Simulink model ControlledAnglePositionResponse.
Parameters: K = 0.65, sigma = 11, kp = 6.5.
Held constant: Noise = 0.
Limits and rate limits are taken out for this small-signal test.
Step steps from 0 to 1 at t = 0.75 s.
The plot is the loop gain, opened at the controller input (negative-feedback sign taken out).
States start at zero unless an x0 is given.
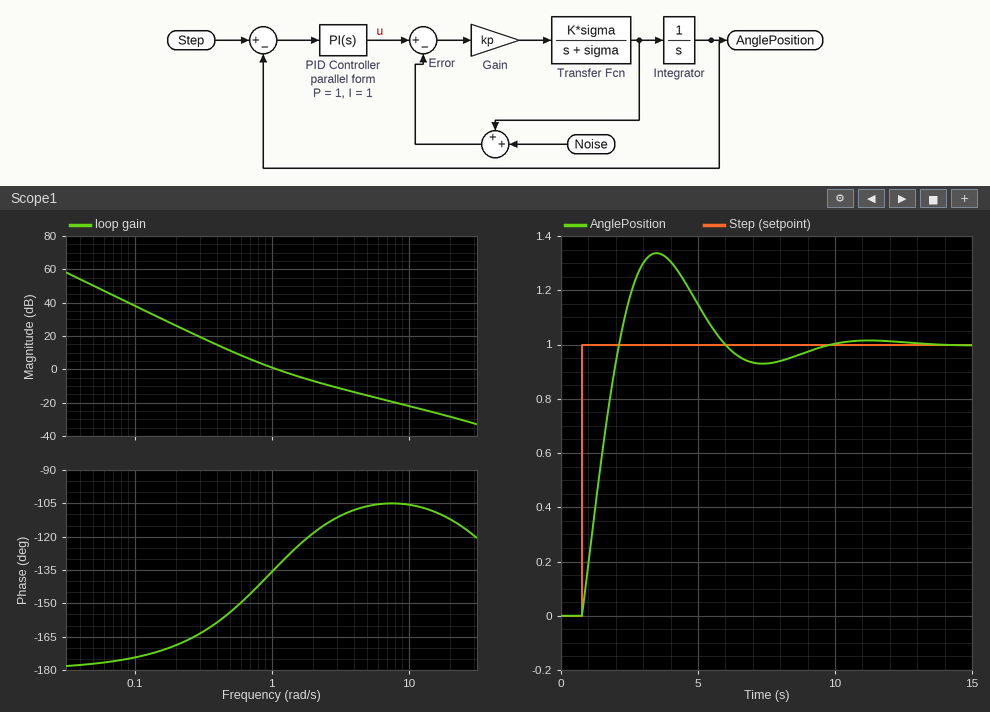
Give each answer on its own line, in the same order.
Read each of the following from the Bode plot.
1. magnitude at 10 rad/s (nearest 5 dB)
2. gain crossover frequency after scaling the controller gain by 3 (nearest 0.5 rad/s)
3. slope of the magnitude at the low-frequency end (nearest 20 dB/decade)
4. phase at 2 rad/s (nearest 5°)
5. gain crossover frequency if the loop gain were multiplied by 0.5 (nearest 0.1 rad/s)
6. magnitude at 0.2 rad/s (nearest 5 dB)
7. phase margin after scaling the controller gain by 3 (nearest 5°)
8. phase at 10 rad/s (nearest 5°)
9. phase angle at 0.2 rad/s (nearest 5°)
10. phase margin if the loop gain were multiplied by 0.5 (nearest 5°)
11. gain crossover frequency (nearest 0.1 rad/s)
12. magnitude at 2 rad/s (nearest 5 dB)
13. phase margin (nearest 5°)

-20 dB
2.5 rad/s
-40 dB/decade
-120°
0.7 rad/s
25 dB
65°
-105°
-170°
35°
1.1 rad/s
-5 dB
45°
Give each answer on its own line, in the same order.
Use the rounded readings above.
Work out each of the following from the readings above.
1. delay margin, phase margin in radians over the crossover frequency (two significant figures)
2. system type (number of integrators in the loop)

0.71 s
2
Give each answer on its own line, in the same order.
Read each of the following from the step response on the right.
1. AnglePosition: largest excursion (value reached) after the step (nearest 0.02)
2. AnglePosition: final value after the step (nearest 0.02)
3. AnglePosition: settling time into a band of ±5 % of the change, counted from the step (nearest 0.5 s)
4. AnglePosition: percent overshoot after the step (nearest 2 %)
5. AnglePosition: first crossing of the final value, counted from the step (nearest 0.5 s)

1.34
1.00
7.5 s
34 %
1.5 s
